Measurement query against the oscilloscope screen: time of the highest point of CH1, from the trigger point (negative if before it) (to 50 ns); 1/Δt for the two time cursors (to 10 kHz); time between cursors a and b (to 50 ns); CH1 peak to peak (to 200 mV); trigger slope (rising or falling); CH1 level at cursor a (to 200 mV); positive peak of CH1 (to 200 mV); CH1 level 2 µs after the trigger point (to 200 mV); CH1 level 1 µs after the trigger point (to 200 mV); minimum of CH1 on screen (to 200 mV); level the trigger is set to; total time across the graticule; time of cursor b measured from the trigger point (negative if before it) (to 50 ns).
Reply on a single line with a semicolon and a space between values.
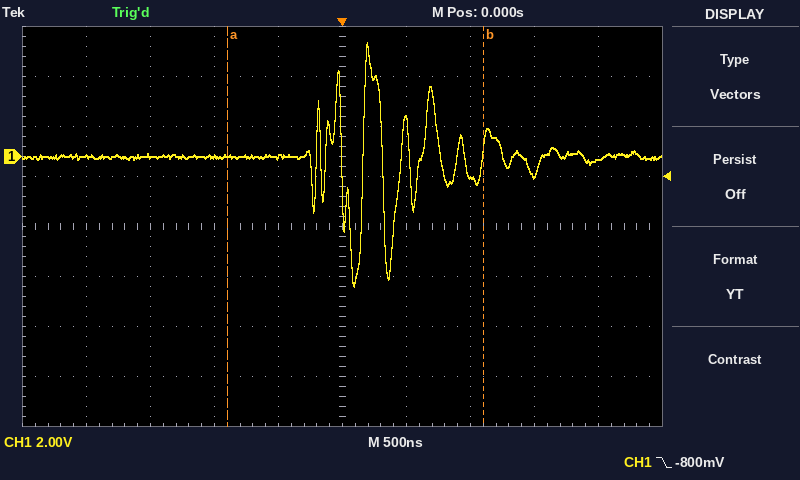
+200 ns; 500 kHz; 2.00 µs; 9.8 V; falling; 0.0 V; 4.6 V; -200 mV; -800 mV; -5.2 V; -800 mV; 5 µs; +1.10 µs
